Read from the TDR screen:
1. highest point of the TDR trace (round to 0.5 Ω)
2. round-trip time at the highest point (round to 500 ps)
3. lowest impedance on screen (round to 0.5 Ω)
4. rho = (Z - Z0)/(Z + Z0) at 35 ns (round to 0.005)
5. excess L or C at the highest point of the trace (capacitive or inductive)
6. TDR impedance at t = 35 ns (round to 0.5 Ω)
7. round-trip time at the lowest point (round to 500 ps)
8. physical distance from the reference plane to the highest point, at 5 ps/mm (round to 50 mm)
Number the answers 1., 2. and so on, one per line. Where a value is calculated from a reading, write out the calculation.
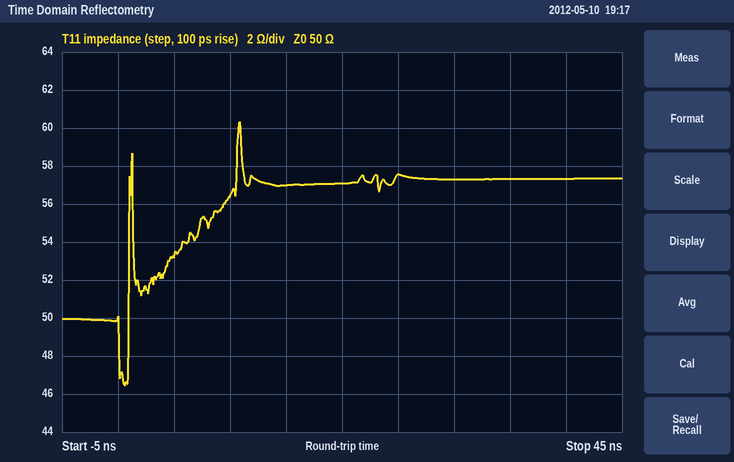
1. 60.5 Ω
2. 11.0 ns
3. 46.5 Ω
4. (57.5 − 50)/(57.5 + 50) ≈ +0.070
5. inductive
6. 57.5 Ω
7. 500 ps
8. 11.0 ns / 2 / 5 ps/mm ≈ 1.10 m
